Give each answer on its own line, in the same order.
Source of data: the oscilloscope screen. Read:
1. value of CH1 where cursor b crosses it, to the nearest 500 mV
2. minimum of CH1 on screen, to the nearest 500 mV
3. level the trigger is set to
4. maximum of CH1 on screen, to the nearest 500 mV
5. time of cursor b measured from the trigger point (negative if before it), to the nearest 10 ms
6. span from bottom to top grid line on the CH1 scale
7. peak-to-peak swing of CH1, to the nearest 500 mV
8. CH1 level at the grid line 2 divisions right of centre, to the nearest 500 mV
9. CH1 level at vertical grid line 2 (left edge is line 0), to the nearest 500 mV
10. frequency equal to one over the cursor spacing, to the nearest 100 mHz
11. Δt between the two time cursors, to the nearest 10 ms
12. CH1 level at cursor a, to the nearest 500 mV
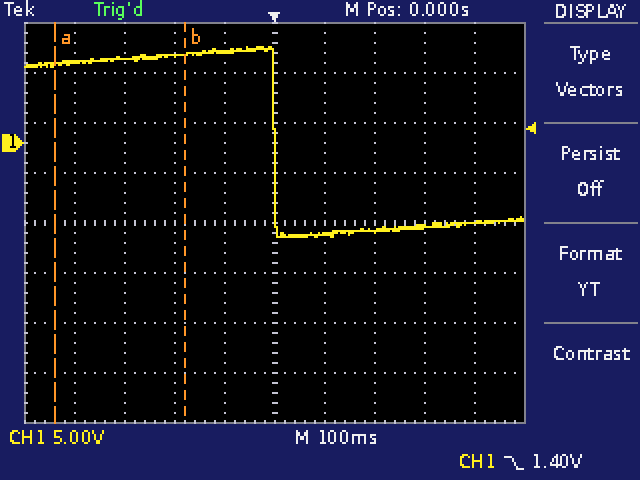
9.0 V
-9.5 V
1.40 V
9.5 V
-180 ms
40 V
19.0 V
-9.0 V
8.5 V
3.8 Hz
260 ms
8.0 V
